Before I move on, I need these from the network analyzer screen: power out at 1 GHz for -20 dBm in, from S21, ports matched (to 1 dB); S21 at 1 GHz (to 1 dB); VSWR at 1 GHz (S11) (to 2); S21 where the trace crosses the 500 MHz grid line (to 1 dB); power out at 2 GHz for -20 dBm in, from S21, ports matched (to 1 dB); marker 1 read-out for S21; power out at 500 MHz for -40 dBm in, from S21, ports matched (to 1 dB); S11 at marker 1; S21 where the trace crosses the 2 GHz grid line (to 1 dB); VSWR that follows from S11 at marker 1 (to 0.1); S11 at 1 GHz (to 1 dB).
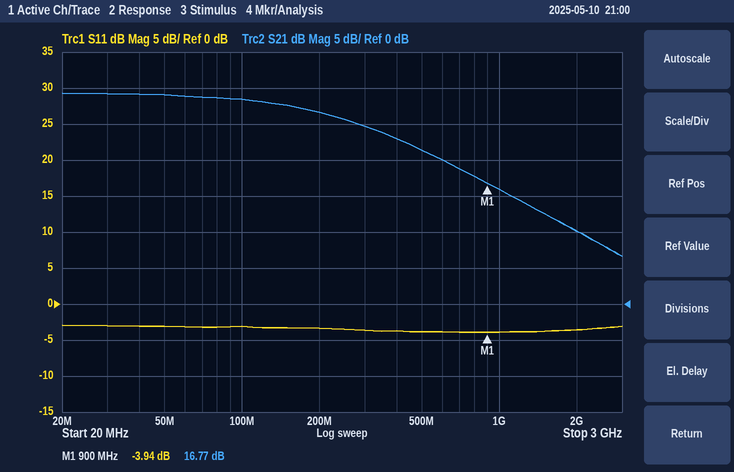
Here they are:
-4 dBm
16 dB
4
21 dB
-10 dBm
16.77 dB
-19 dBm
-3.94 dB
10 dB
4.5
-4 dB
